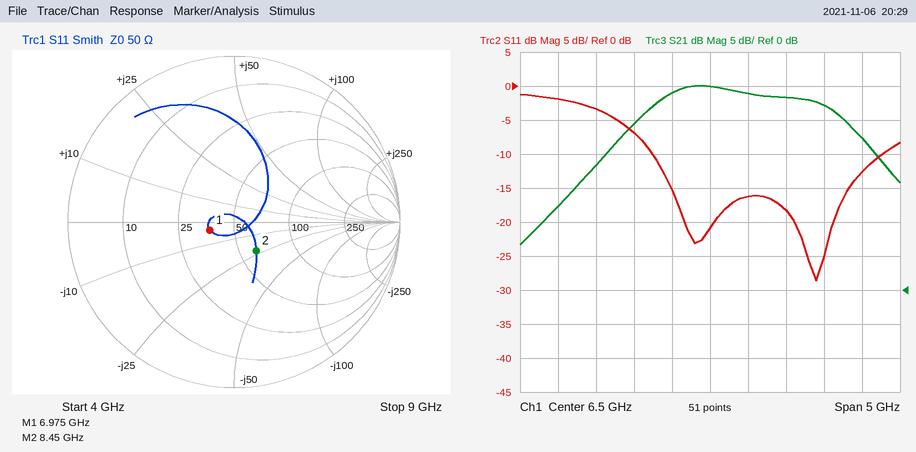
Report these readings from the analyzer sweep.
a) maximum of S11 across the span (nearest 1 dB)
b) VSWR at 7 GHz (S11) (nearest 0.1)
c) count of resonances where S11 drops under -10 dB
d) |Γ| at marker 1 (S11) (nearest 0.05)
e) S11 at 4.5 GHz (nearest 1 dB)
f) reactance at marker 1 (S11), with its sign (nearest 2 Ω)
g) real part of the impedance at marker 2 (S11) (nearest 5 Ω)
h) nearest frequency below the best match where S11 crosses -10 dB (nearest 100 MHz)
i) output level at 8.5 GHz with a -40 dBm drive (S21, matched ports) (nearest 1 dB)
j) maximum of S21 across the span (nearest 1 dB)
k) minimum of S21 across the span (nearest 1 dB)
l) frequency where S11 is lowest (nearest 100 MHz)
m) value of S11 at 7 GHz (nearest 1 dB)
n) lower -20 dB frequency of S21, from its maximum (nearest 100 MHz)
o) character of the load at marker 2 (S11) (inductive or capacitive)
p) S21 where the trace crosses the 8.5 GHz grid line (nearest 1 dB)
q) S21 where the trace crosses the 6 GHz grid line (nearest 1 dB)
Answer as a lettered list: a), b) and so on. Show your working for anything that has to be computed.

a) -1 dB
b) |Γ| = 10^(-16/20) = 0.1585; VSWR = (1 + 0.1585)/(1 − 0.1585) ≈ 1.4
c) 2
d) 0.15
e) -2 dB
f) -4 Ω
g) 60 Ω
h) 5.7 GHz
i) -40 dBm + (22 dB) = -18 dBm
j) 30 dB
k) 7 dB
l) 7.9 GHz
m) -16 dB
n) 4.3 GHz
o) capacitive
p) 22 dB
q) 29 dB
